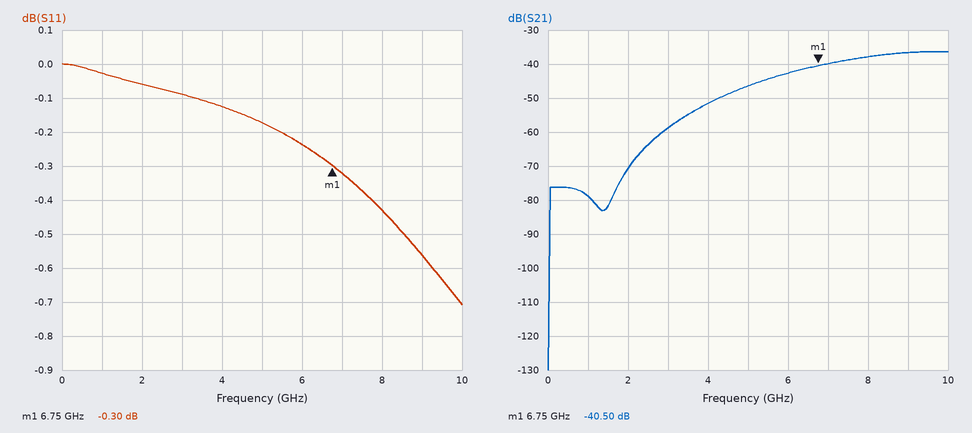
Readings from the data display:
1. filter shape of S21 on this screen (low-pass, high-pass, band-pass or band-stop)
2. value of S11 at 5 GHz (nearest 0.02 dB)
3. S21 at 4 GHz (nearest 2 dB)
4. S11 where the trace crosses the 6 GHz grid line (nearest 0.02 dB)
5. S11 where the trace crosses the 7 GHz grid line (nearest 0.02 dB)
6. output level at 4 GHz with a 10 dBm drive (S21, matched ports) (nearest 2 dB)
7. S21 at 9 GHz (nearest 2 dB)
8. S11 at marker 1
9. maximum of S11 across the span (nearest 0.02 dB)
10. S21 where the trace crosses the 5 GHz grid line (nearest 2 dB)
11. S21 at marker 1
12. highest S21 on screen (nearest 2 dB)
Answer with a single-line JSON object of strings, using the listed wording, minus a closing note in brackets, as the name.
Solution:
{"filter shape of S21 on this screen": "high-pass", "value of S11 at 5 GHz": "-0.18 dB", "S21 at 4 GHz": "-52 dB", "S11 where the trace crosses the 6 GHz grid line": "-0.24 dB", "S11 where the trace crosses the 7 GHz grid line": "-0.32 dB", "output level at 4 GHz with a 10 dBm drive (S21, matched ports)": "-42 dBm", "S21 at 9 GHz": "-36 dB", "S11 at marker 1": "-0.30 dB", "maximum of S11 across the span": "0.00 dB", "S21 where the trace crosses the 5 GHz grid line": "-46 dB", "S21 at marker 1": "-40.50 dB", "highest S21 on screen": "-36 dB"}
